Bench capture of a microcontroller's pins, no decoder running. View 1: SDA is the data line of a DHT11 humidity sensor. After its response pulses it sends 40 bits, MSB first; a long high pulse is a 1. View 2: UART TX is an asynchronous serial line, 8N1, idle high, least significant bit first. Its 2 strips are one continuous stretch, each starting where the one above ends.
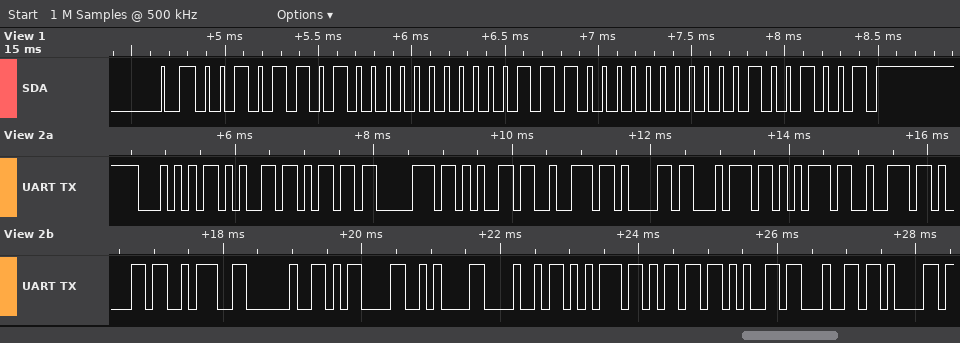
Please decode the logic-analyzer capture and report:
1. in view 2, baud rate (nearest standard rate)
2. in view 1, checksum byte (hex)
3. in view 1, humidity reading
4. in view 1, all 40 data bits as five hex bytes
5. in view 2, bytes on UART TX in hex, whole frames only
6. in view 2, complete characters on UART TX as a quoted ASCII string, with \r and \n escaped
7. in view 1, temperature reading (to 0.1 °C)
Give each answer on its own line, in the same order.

9600 baud
0x49
45 %
2D 00 1C 00 49
54 65 6D 70 65 72 61 74 75 72 61 3A 20 0D 0A 48 75 6D 65 64 61
"Temperatura: \r\nHumeda"
28.0 °C
